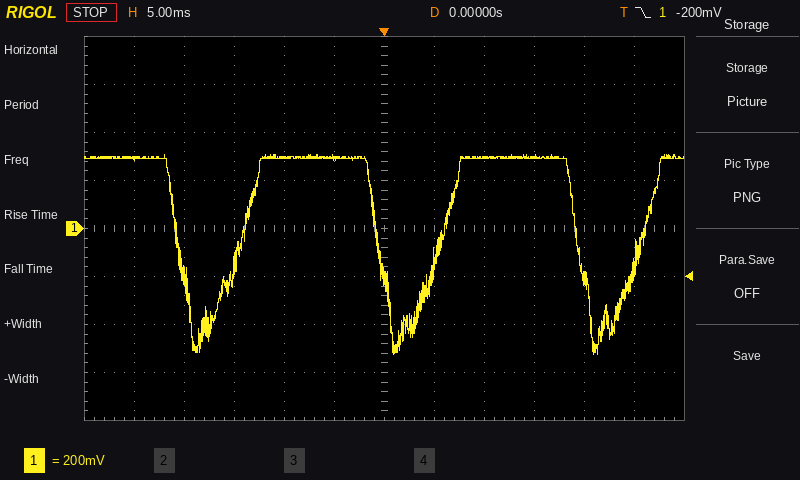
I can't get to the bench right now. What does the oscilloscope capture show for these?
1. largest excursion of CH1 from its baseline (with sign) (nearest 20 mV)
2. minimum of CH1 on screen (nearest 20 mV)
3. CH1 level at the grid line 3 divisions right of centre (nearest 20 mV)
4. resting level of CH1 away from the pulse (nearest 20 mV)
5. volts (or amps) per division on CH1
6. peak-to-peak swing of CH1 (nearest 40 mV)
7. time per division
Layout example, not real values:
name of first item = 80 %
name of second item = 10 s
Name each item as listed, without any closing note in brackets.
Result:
largest excursion of CH1 from its baseline (with sign) = -820 mV
minimum of CH1 on screen = -520 mV
CH1 level at the grid line 3 divisions right of centre = 300 mV
resting level of CH1 away from the pulse = 300 mV
volts (or amps) per division on CH1 = 200 mV
peak-to-peak swing of CH1 = 840 mV
time per division = 5 ms
